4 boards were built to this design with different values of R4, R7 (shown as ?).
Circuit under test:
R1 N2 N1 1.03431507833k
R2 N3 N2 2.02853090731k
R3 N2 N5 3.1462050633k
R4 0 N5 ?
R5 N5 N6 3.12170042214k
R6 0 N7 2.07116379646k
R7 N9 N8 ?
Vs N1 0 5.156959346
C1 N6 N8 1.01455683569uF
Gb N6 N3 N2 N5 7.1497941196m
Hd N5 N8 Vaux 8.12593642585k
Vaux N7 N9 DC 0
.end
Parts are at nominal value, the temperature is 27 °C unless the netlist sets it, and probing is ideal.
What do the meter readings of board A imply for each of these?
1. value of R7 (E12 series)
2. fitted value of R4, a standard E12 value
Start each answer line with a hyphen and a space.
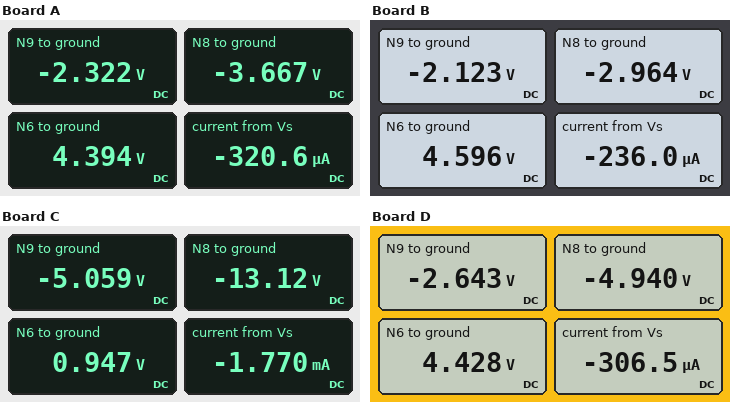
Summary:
- 1.2 kΩ
- 6.8 kΩ
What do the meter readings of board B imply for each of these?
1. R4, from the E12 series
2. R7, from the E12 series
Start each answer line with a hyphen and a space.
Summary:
- 6.8 kΩ
- 820 Ω
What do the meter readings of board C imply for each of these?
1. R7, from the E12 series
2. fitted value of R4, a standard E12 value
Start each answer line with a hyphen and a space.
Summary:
- 3.3 kΩ
- 10 kΩ
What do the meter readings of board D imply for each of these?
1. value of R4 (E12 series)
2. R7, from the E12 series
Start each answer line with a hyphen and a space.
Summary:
- 5.6 kΩ
- 1.8 kΩ
